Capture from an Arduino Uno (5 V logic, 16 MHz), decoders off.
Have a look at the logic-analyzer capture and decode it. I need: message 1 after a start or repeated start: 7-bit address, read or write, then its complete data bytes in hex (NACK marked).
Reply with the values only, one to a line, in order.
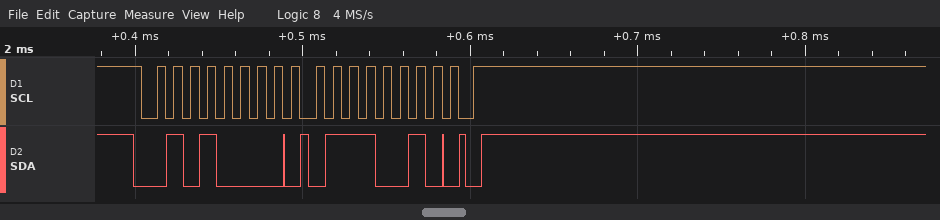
0x28 write: 72
